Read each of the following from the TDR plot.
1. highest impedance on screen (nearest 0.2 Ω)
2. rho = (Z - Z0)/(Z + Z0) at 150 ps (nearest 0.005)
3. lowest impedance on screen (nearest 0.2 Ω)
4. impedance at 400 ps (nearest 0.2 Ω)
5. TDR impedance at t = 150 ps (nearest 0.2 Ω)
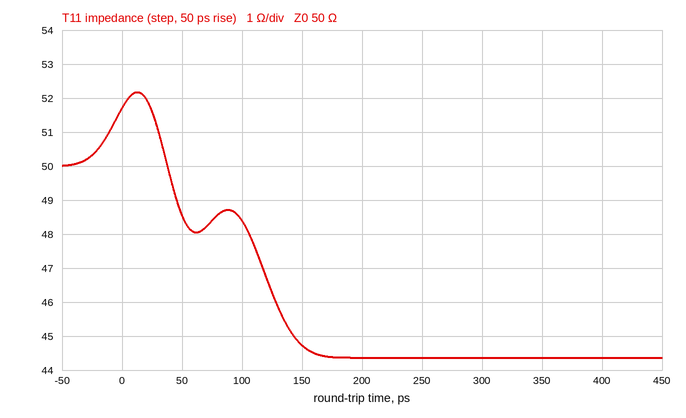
52.2 Ω
-0.055
44.4 Ω
44.4 Ω
44.8 Ω
